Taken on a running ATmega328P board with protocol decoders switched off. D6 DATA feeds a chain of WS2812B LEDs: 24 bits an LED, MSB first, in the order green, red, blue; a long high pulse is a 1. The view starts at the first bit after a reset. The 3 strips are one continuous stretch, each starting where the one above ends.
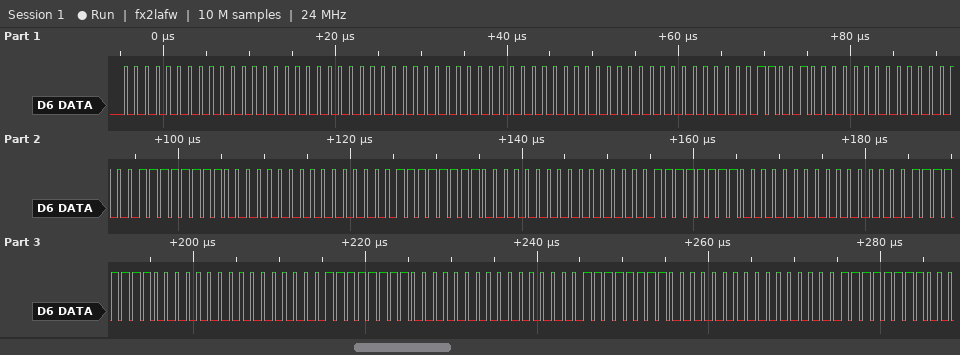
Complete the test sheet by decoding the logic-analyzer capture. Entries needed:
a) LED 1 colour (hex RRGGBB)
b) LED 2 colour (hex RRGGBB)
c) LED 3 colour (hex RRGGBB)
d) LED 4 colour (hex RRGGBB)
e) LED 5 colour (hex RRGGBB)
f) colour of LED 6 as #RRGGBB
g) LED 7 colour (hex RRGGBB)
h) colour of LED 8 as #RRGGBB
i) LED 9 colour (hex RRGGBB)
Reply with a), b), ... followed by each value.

a) #000000
b) #000000
c) #190000
d) #FF0000
e) #FF0000
f) #FF0000
g) #FF0000
h) #FF0000
i) #FF0000
